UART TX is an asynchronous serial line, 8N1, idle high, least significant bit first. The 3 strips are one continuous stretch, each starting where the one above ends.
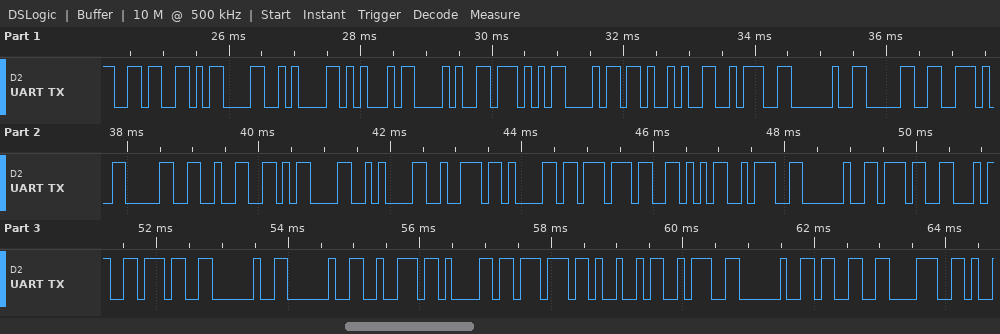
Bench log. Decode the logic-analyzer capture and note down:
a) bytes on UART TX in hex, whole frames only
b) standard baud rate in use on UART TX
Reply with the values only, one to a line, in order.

0x36 0x0D 0x0A 0x45 0x28 0x57 0x68 0x29 0x3A 0x20 0x30 0x2E 0x30 0x32 0x0D 0x0A 0x72 0x61 0x77 0x56 0x3A 0x20 0x37 0x34 0x37 0x20 0x20 0x72 0x61 0x77 0x49 0x3A 0x20 0x33 0x38
9600 baud
